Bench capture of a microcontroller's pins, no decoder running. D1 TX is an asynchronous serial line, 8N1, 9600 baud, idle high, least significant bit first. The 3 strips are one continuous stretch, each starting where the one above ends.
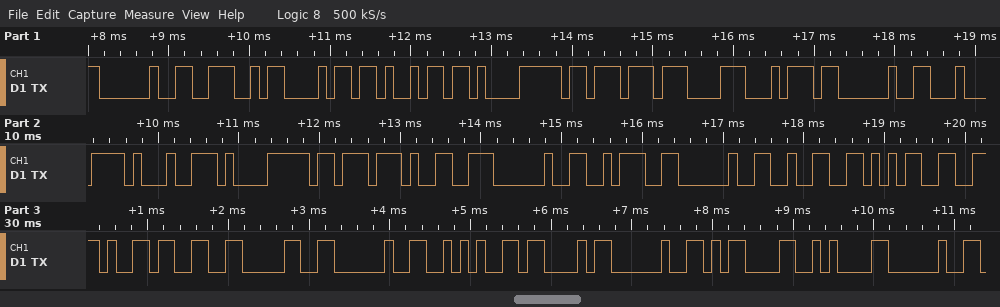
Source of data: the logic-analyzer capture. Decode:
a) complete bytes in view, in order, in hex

20 4E 68 69 E1 BB 87 74 20 C4 91 E1 BB 99 20 3A 20 32 35 2E 33 30 20 2A 43 20 0D 0A 20
